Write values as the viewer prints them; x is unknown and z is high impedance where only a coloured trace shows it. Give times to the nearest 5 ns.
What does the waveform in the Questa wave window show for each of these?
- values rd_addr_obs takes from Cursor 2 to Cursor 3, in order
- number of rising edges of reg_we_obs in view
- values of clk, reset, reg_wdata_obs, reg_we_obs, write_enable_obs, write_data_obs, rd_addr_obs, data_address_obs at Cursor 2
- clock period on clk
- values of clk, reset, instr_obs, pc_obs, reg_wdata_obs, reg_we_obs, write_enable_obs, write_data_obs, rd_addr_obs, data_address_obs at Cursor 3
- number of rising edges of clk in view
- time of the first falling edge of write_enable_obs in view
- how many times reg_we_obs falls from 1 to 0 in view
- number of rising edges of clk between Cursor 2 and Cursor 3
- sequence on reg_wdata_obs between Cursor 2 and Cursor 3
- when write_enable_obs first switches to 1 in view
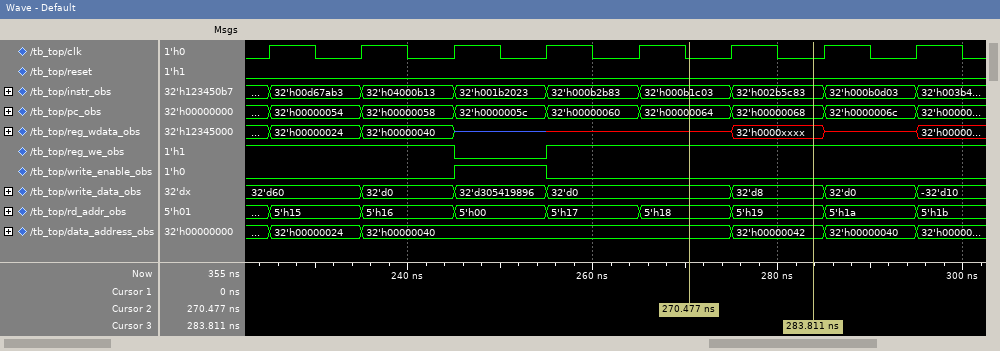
5'h18, 5'h19
1
clk=0, reset=0, reg_wdata_obs=x, reg_we_obs=1, write_enable_obs=0, write_data_obs=32'd0, rd_addr_obs=5'h18, data_address_obs=32'h00000040
10 ns
clk=0, reset=0, instr_obs=32'h002b5c83, pc_obs=32'h00000068, reg_wdata_obs=32'h0000xxxx, reg_we_obs=1, write_enable_obs=0, write_data_obs=32'd8, rd_addr_obs=5'h19, data_address_obs=32'h00000042
8
255 ns
1
1
x, 32'h0000xxxx
245 ns
